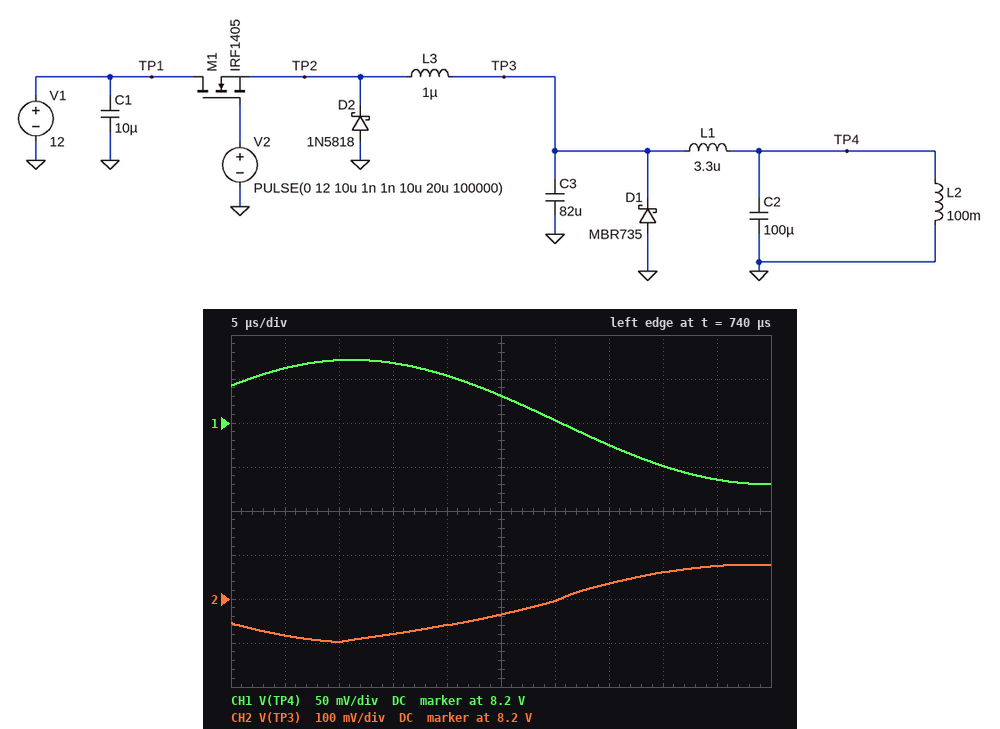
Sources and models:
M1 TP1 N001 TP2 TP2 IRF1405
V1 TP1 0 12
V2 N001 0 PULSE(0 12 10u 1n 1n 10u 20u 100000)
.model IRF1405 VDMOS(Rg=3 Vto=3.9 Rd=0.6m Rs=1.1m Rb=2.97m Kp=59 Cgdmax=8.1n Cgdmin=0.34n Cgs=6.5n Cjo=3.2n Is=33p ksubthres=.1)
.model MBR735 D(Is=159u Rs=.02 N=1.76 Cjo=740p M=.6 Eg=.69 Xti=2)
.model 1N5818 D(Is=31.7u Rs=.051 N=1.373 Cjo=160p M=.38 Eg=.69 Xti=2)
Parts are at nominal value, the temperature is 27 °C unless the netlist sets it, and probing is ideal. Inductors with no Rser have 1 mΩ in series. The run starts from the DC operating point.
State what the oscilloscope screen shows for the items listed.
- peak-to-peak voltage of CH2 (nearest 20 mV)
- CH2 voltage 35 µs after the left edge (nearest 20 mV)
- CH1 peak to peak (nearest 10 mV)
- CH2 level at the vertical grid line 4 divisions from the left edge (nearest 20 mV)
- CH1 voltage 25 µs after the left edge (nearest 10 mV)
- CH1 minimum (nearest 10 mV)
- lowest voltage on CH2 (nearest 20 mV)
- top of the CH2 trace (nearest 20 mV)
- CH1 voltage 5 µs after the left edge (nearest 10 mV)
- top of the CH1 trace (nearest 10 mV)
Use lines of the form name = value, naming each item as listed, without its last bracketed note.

peak-to-peak voltage of CH2 = 180 mV
CH2 voltage 35 µs after the left edge = 8.24 V
CH1 peak to peak = 140 mV
CH2 level at the vertical grid line 4 divisions from the left edge = 8.14 V
CH1 voltage 25 µs after the left edge = 8.23 V
CH1 minimum = 8.13 V
lowest voltage on CH2 = 8.10 V
top of the CH2 trace = 8.28 V
CH1 voltage 5 µs after the left edge = 8.26 V
top of the CH1 trace = 8.27 V
